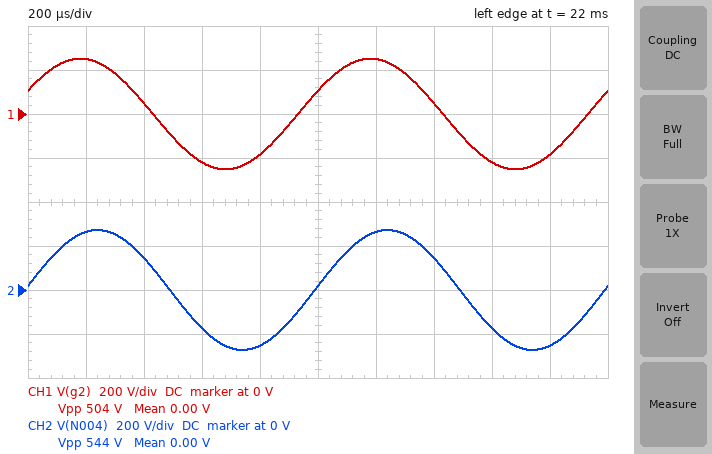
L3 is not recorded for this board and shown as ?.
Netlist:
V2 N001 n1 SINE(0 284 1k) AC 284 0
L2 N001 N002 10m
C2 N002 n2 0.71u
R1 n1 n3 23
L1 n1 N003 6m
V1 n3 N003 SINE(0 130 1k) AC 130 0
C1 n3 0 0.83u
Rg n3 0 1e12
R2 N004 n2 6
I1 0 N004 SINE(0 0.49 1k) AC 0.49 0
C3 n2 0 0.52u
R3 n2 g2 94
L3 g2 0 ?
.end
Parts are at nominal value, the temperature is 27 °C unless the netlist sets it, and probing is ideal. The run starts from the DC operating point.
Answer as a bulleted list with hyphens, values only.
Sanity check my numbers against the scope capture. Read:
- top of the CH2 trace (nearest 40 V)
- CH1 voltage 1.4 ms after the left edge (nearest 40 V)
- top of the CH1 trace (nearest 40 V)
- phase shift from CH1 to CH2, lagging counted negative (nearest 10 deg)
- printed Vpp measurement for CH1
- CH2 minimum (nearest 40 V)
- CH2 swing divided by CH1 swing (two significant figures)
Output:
- 280 V
- 40 V
- 240 V
- -20 deg
- 504 V
- -280 V
- 1.1
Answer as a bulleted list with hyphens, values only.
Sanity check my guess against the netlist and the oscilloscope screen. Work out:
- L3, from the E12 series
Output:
- 39 mH
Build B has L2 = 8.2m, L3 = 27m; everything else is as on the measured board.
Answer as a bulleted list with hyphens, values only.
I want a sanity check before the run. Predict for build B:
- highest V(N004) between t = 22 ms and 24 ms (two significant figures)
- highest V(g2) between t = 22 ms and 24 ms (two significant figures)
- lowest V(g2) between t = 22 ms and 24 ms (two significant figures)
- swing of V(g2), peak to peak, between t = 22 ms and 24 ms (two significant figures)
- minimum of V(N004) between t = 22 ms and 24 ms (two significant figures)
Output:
- 260 V
- 230 V
- -230 V
- 450 V
- -260 V
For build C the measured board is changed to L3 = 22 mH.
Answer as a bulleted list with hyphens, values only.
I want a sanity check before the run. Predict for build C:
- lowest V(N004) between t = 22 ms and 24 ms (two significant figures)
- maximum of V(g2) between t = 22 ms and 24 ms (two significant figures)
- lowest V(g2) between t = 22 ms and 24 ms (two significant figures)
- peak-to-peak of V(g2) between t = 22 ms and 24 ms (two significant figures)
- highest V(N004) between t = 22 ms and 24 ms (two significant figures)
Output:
- -220 V
- 180 V
- -180 V
- 360 V
- 220 V
